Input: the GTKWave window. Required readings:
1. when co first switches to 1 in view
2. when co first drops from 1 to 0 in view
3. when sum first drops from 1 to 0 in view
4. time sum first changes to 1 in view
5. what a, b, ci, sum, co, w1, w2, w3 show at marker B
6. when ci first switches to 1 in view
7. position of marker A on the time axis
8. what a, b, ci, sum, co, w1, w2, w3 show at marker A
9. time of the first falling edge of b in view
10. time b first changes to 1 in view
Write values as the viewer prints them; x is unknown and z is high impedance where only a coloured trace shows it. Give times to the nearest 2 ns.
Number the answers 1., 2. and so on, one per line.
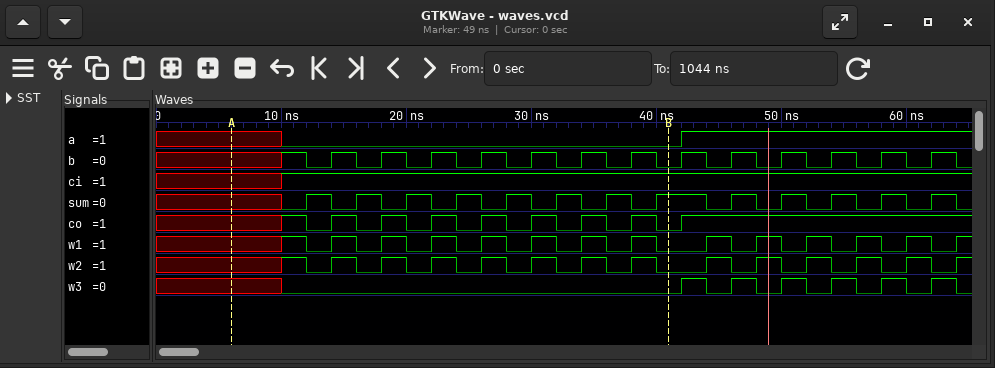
1. 10 ns
2. 12 ns
3. 14 ns
4. 12 ns
5. a=0, b=0, ci=1, sum=1, co=0, w1=0, w2=0, w3=0
6. 10 ns
7. 6 ns
8. a=x, b=x, ci=x, sum=x, co=x, w1=x, w2=x, w3=x
9. 12 ns
10. 10 ns
